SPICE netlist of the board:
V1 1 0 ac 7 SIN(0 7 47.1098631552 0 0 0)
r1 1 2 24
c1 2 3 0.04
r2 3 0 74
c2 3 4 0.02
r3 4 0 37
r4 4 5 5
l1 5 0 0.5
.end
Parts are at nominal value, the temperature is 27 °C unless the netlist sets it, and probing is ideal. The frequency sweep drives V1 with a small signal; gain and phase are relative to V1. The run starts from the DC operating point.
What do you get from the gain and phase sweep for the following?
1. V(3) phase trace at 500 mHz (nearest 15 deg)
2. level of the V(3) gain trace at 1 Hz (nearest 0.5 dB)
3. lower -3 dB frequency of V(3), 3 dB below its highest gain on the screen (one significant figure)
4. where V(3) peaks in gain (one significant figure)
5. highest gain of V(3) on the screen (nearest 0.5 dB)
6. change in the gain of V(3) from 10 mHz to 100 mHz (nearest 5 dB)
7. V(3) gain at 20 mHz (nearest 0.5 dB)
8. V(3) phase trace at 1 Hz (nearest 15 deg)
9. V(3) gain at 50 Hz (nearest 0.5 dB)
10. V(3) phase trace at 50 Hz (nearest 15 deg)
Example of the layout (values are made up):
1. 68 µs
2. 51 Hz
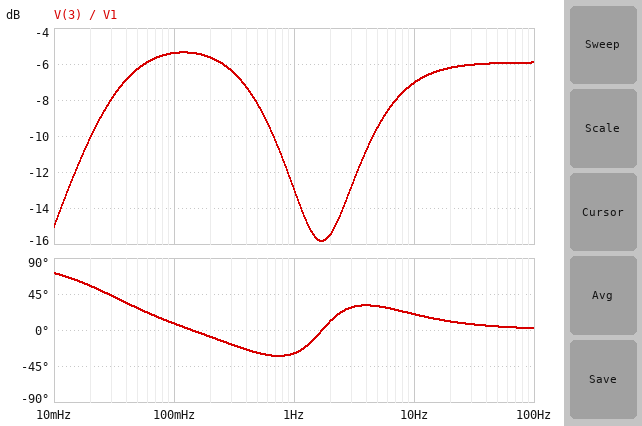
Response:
1. -30 deg
2. -13.0 dB
3. 30 mHz
4. 100 mHz
5. -5.5 dB
6. 10 dB
7. -10.0 dB
8. -30 deg
9. -6.0 dB
10. 0 deg
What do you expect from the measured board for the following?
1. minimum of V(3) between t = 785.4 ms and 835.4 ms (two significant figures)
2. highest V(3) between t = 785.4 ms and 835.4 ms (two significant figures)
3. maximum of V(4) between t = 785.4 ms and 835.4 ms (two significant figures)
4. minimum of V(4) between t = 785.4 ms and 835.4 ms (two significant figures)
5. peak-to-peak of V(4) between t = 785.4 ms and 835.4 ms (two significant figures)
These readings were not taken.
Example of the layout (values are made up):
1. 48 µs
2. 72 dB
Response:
1. -3.5 V
2. 3.5 V
3. 3.5 V
4. -3.5 V
5. 7.1 V
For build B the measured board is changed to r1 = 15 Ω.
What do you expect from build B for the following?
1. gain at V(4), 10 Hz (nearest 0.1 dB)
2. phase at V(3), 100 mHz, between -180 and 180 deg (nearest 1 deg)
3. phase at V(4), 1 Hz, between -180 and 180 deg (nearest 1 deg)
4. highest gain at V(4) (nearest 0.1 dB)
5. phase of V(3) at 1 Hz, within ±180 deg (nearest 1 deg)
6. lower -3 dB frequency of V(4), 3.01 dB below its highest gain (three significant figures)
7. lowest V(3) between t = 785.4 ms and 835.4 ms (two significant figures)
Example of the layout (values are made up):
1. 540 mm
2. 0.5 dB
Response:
1. -4.7 dB
2. 12 deg
3. 56 deg
4. -4.1 dB
5. -22 deg
6. 3.56 Hz
7. -4.3 V
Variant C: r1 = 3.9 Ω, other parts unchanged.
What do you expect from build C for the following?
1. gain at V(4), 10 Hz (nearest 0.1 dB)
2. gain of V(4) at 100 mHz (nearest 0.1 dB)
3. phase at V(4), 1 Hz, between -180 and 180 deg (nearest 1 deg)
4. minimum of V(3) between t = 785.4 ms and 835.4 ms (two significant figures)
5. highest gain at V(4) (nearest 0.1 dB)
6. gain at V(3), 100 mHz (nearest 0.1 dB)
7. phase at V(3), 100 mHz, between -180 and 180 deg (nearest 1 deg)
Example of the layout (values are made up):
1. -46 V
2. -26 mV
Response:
1. -1.2 dB
2. -29.4 dB
3. 78 deg
4. -6.0 V
5. -1.1 dB
6. -4.3 dB
7. 18 deg
